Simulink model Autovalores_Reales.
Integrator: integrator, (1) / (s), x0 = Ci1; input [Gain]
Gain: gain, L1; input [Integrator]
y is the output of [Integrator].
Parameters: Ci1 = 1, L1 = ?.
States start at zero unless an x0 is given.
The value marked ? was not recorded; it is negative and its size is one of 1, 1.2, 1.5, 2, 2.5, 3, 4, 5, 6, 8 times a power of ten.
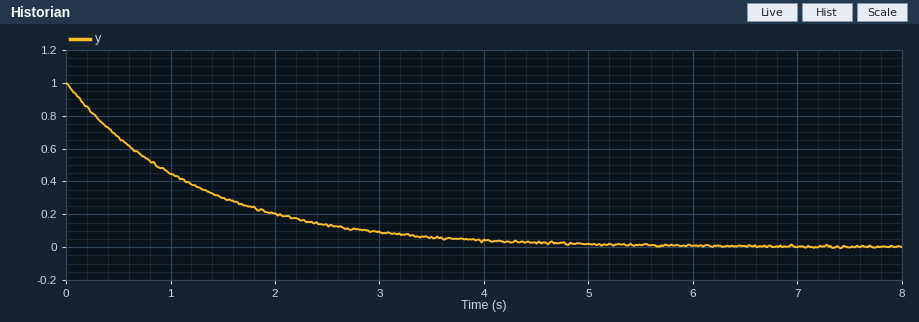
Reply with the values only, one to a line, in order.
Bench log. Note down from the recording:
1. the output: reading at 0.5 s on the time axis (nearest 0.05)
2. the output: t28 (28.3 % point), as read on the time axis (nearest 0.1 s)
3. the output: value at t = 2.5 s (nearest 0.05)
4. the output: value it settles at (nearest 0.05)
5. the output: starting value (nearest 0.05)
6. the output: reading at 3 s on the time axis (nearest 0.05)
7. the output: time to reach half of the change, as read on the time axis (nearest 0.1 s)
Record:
0.65
0.4 s
0.15
0.00
1.00
0.10
0.9 s
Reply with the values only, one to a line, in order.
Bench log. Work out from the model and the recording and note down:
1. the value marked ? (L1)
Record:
-0.8
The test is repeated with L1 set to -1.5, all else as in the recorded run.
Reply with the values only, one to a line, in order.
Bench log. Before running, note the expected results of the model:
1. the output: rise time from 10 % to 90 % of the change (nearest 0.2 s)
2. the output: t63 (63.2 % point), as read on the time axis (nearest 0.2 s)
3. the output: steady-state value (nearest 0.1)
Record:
1.4 s
0.6 s
0.0
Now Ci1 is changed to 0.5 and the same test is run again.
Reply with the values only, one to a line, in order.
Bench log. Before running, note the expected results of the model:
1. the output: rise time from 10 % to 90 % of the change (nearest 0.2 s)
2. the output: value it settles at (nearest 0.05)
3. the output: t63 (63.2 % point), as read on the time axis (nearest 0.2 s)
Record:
2.8 s
0.00
1.2 s
